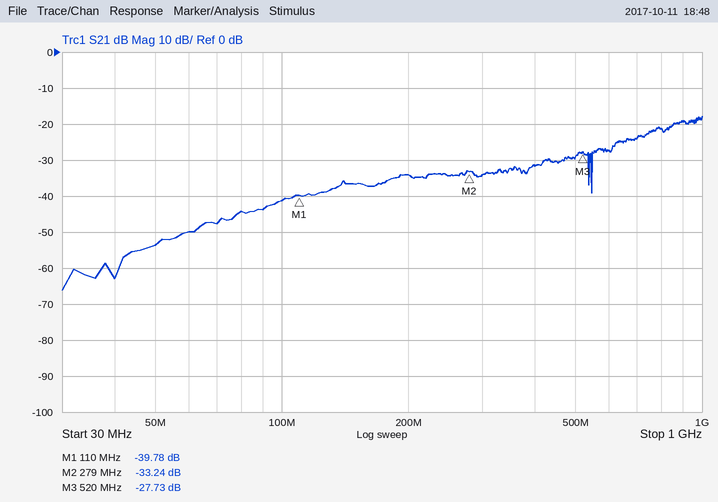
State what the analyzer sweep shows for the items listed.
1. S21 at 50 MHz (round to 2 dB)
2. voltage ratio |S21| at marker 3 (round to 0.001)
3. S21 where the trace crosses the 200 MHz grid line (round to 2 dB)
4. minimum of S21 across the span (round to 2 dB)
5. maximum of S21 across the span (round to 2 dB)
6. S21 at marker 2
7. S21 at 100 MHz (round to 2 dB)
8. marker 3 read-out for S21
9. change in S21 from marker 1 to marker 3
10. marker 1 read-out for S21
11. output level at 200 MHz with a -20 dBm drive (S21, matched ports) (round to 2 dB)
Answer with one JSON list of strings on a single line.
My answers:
["-54 dB", "0.041", "-34 dB", "-66 dB", "-18 dB", "-33.24 dB", "-42 dB", "-27.73 dB", "12.05 dB", "-39.78 dB", "-54 dBm"]
